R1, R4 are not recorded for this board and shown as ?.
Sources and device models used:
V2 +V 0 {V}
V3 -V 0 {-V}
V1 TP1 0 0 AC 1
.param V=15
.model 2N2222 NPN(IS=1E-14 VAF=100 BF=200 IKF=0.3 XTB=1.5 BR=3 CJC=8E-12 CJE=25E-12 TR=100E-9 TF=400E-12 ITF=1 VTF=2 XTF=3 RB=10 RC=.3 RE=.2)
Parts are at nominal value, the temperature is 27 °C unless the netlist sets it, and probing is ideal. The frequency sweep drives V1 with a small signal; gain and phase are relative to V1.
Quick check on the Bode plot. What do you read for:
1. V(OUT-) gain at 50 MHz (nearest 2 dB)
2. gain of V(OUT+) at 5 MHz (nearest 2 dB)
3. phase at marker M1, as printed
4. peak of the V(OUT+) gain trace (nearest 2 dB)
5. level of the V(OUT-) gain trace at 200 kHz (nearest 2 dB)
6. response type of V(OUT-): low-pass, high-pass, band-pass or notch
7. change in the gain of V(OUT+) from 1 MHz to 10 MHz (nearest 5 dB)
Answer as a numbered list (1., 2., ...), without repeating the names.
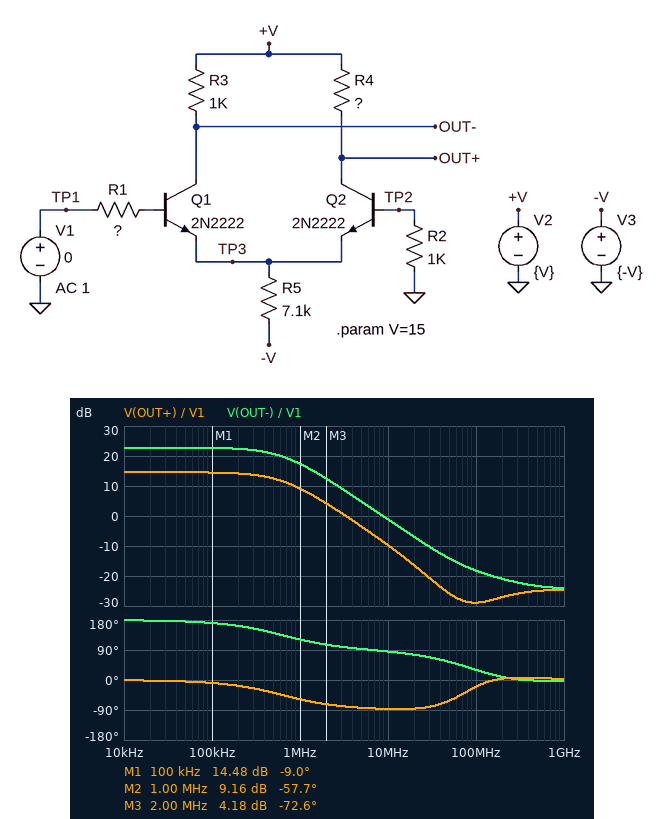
1. -14 dB
2. -4 dB
3. -9.0 deg
4. 14 dB
5. 22 dB
6. low-pass
7. -20 dB
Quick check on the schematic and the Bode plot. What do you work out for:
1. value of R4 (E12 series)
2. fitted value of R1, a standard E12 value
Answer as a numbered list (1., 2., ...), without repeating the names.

1. 390 Ω
2. 3.3 kΩ
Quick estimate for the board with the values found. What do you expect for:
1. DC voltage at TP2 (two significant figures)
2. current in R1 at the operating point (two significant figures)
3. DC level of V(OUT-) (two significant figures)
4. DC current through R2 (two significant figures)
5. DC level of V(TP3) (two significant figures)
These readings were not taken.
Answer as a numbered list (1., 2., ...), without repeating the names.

1. -5.0 mV
2. 3.8 µA
3. 14 V
4. 5.0 µA
5. -660 mV
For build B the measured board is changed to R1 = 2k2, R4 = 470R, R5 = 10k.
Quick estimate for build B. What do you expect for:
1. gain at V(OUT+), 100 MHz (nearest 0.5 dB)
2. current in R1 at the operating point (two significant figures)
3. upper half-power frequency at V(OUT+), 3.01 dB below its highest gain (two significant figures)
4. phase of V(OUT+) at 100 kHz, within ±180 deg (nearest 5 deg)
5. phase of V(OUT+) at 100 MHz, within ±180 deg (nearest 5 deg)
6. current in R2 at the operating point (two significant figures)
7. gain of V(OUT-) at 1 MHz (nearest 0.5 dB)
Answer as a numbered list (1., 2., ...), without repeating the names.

1. -25.0 dB
2. 2.9 µA
3. 960 kHz
4. -5 deg
5. -10 deg
6. 3.3 µA
7. 18.0 dB
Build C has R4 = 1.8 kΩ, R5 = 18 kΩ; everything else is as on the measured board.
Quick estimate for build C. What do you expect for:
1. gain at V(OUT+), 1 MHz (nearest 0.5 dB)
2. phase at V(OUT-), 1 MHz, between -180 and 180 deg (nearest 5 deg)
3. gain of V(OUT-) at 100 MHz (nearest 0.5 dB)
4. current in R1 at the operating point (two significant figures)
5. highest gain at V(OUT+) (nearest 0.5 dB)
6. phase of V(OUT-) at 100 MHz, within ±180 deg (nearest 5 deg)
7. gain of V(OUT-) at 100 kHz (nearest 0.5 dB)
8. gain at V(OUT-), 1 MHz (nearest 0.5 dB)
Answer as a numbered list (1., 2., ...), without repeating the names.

1. 17.5 dB
2. 130 deg
3. -18.0 dB
4. 1.6 µA
5. 21.5 dB
6. 20 deg
7. 16.5 dB
8. 12.5 dB
